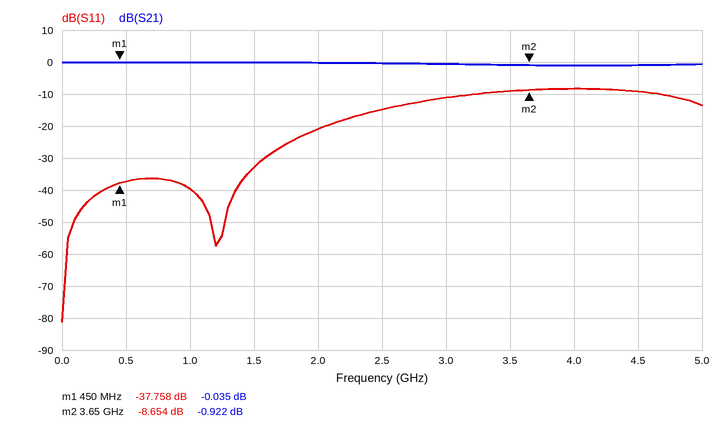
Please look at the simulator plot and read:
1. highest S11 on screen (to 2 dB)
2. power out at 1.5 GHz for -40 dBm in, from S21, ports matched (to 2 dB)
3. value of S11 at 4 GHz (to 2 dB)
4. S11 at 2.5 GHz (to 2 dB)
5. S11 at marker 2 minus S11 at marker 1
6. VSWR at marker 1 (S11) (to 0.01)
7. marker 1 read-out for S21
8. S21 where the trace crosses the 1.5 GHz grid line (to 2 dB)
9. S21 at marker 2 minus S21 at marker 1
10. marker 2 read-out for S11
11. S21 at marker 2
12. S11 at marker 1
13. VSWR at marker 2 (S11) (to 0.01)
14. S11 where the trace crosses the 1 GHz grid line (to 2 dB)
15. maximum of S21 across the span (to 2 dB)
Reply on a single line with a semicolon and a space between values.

-8 dB; -40 dBm; -8 dB; -14 dB; 29.104 dB; 1.03; -0.035 dB; 0 dB; -0.887 dB; -8.654 dB; -0.922 dB; -37.758 dB; 2.17; -40 dB; 0 dB
